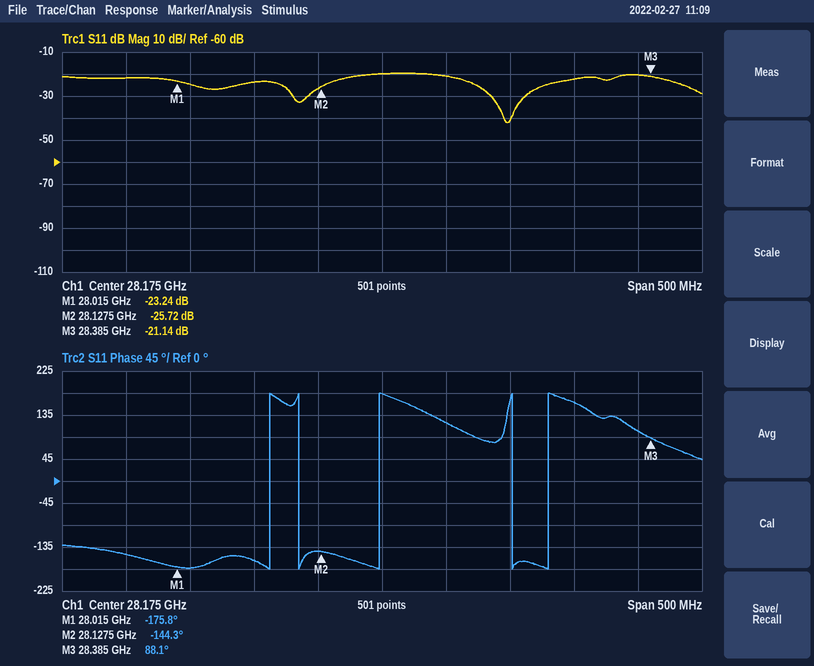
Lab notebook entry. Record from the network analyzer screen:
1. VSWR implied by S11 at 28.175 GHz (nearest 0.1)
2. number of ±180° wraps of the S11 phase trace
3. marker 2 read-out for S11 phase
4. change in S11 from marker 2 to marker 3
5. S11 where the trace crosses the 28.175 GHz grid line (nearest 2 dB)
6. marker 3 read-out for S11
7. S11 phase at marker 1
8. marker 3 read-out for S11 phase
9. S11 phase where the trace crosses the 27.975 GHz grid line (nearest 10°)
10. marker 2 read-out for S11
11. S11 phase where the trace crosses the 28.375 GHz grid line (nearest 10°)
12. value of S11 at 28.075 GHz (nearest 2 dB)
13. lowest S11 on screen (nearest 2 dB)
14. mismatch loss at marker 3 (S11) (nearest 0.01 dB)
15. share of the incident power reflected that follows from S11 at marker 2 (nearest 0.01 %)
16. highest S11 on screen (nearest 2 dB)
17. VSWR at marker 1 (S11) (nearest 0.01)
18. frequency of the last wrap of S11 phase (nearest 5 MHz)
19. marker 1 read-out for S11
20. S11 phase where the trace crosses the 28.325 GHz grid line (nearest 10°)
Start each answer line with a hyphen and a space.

- 1.2
- 5
- -144.3°
- 4.58 dB
- -20 dB
- -21.14 dB
- -175.8°
- 88.1°
- -150°
- -25.72 dB
- 100°
- -24 dB
- -42 dB
- 0.03 dB
- 0.27 %
- -20 dB
- 1.15
- 28.305 GHz
- -23.24 dB
- 160°
